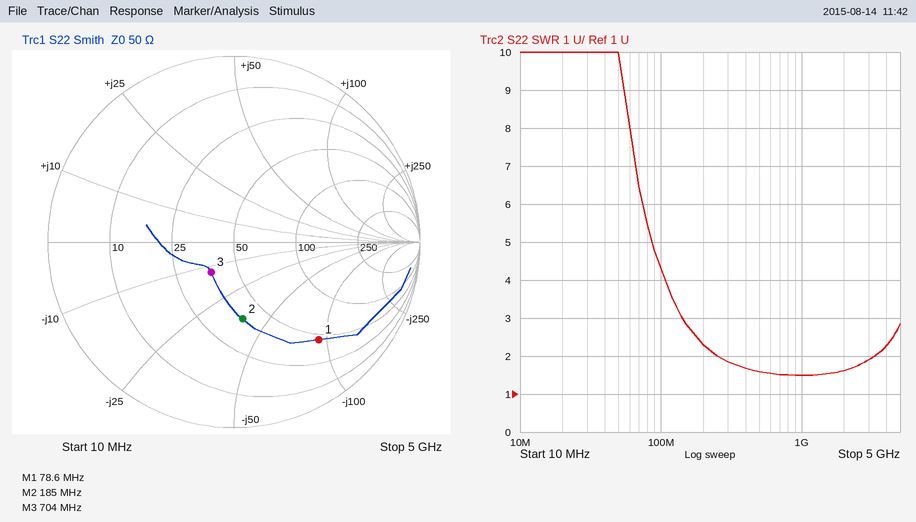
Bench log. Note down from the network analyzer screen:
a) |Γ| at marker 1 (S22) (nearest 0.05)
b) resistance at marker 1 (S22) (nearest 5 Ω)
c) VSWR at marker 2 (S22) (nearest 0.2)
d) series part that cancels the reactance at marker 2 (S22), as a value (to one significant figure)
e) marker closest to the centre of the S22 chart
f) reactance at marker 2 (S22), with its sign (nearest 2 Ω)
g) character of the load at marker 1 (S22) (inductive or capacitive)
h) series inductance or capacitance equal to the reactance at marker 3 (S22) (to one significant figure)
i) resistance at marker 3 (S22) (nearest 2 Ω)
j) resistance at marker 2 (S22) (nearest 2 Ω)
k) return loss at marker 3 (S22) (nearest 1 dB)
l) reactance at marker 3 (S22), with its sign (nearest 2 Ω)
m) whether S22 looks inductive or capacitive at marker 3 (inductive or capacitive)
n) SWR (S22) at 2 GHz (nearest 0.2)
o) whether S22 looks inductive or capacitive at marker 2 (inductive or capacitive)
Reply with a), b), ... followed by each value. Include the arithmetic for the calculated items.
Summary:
a) 0.70
b) 45 Ω
c) 2.4
d) L = 38 Ω/(2π × 185 MHz) ≈ 32.7 nH, so 30 nH to one significant figure
e) marker 3
f) -38 Ω
g) capacitive
h) C = 1/(2π × 704 MHz × 12 Ω) ≈ 18.8 pF, so 20 pF to one significant figure
i) 38 Ω
j) 38 Ω
k) 14 dB
l) -12 Ω
m) capacitive
n) 1.6
o) capacitive
